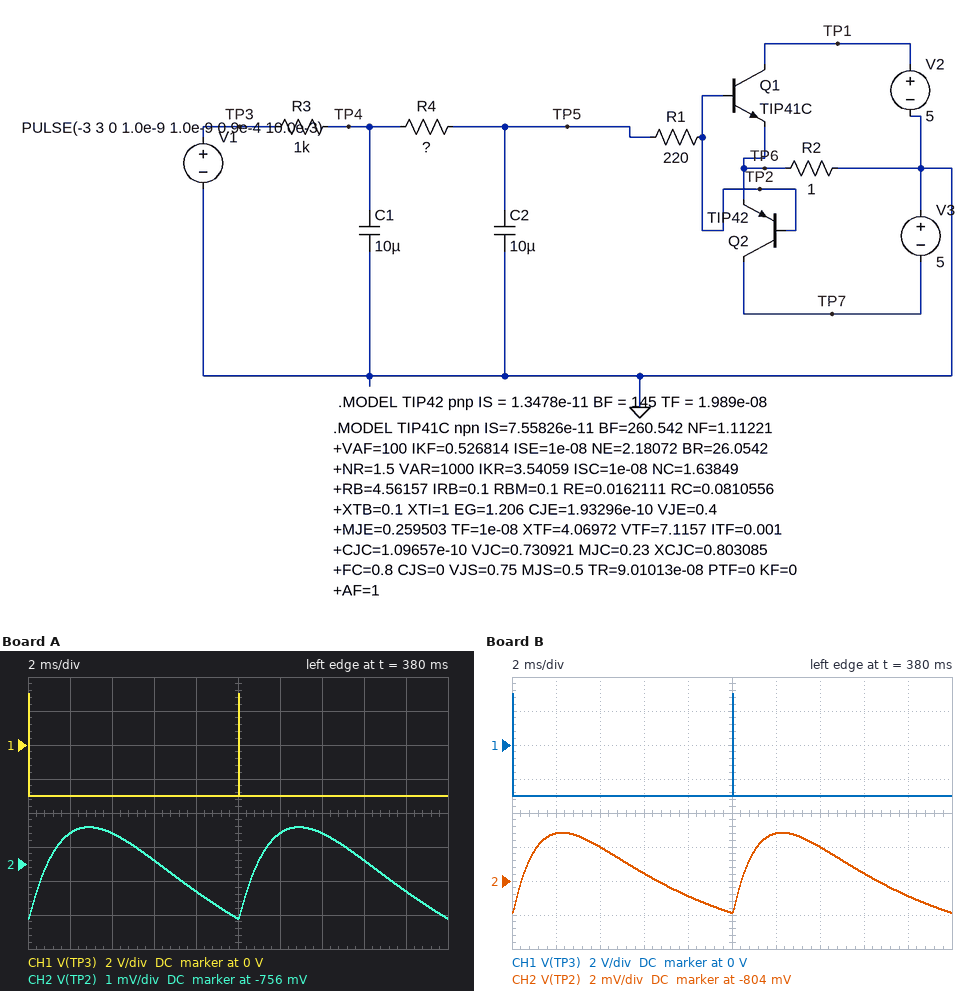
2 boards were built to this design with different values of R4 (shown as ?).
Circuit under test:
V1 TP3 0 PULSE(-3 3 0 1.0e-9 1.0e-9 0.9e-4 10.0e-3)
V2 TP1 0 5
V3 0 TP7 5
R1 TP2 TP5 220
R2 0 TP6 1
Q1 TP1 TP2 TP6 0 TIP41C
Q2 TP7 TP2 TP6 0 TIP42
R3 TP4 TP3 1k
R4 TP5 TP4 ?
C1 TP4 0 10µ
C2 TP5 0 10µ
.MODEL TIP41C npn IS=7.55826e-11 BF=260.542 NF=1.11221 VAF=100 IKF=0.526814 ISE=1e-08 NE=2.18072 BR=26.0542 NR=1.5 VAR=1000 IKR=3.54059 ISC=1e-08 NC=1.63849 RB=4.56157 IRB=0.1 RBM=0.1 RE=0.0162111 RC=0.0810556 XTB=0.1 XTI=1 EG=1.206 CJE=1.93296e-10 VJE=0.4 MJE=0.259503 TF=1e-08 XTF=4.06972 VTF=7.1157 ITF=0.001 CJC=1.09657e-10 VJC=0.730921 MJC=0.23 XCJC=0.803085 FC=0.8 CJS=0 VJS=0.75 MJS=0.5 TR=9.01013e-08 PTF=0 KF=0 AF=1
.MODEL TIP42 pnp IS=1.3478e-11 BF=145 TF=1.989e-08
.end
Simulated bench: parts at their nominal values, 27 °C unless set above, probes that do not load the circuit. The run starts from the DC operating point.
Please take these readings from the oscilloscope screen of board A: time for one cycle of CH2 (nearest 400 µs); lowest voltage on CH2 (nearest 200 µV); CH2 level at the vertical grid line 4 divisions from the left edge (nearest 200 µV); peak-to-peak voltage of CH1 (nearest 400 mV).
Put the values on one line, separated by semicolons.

10.0 ms; -757.6 mV; -756.8 mV; 6.0 V
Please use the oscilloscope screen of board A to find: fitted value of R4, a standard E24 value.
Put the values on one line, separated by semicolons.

820 Ω
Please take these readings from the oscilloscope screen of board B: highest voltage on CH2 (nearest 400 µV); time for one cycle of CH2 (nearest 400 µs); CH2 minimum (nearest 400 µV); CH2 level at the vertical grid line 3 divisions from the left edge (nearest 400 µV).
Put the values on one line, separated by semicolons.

-801.2 mV; 10.0 ms; -806.0 mV; -803.6 mV
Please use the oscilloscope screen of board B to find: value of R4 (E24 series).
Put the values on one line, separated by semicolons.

360 Ω
